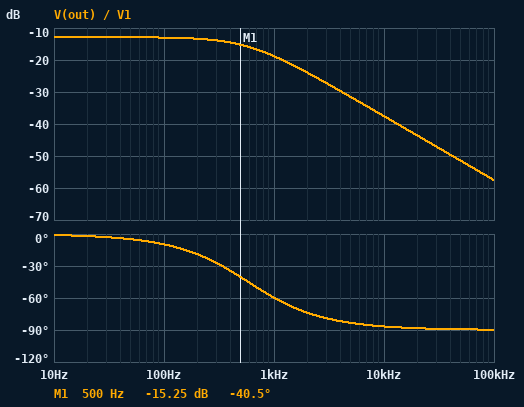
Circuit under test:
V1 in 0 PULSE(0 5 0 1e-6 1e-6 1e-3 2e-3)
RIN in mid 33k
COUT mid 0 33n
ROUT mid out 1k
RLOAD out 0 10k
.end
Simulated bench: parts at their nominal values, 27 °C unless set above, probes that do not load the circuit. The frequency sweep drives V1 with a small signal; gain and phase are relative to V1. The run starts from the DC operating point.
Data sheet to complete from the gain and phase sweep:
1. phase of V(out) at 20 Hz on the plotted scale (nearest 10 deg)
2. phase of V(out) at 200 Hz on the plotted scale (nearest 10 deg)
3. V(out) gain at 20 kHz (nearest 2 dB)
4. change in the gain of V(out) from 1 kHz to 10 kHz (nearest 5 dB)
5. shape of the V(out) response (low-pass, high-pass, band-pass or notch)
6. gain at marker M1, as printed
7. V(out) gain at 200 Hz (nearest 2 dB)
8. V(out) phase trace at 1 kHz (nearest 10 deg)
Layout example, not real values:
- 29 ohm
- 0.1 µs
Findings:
- 0 deg
- -20 deg
- -44 dB
- -20 dB
- low-pass
- -15.25 dB
- -14 dB
- -60 deg
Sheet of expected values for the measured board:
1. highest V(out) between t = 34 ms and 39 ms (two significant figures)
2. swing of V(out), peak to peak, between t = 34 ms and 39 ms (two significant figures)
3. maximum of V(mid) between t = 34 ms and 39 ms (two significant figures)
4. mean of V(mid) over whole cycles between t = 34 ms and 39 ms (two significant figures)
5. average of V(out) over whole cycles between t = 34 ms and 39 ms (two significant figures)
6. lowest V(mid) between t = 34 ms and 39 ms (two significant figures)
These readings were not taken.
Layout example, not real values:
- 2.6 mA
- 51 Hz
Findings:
- 1.1 V
- 1.1 V
- 1.2 V
- 630 mV
- 570 mV
- 31 mV
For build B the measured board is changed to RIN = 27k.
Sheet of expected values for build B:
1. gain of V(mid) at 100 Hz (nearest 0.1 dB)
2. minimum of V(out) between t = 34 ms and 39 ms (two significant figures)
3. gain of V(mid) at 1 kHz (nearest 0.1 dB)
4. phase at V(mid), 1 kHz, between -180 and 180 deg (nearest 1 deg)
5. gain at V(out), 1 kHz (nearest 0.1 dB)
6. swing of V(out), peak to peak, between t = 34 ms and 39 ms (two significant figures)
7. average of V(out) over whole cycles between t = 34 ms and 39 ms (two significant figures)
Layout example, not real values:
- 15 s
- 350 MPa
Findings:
- -10.9 dB
- 27 mV
- -16.4 dB
- -58 deg
- -17.2 dB
- 1.3 V
- 660 mV
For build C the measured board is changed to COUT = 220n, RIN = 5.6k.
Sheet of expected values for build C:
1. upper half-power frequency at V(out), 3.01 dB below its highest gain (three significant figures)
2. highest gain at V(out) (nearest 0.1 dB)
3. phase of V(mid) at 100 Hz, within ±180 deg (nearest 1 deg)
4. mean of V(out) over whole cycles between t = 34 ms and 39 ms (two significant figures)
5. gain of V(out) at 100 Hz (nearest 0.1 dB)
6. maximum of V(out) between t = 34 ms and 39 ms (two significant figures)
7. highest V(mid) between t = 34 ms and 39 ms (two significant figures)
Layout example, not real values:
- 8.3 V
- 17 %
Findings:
- 195 Hz
- -4.4 dB
- -27 deg
- 1.5 V
- -5.4 dB
- 2.3 V
- 2.6 V
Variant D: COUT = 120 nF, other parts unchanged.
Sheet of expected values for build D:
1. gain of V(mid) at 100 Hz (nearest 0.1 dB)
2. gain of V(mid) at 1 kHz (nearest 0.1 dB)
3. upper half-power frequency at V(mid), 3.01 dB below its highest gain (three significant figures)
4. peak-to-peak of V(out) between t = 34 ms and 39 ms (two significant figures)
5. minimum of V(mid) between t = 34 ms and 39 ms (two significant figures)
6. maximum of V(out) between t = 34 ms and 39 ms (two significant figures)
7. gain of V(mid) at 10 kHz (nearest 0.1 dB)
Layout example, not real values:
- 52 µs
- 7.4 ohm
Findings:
- -13.5 dB
- -28.0 dB
- 161 Hz
- 530 mV
- 330 mV
- 830 mV
- -47.9 dB
